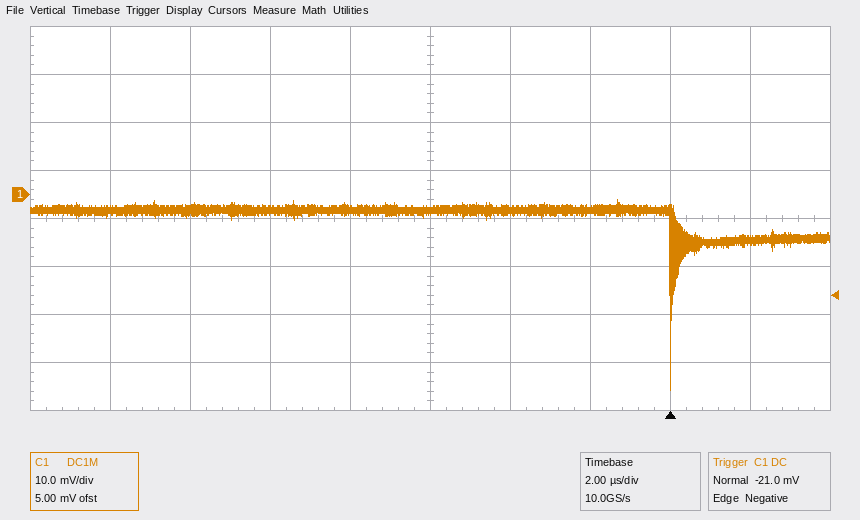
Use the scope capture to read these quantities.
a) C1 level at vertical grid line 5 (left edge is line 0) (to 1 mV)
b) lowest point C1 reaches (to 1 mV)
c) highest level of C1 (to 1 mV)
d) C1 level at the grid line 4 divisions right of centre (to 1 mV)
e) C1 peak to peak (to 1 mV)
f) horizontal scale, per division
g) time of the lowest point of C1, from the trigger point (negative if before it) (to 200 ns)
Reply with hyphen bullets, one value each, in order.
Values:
- -3 mV
- -41 mV
- -1 mV
- -10 mV
- 40 mV
- 2 µs
- 0.0 µs
